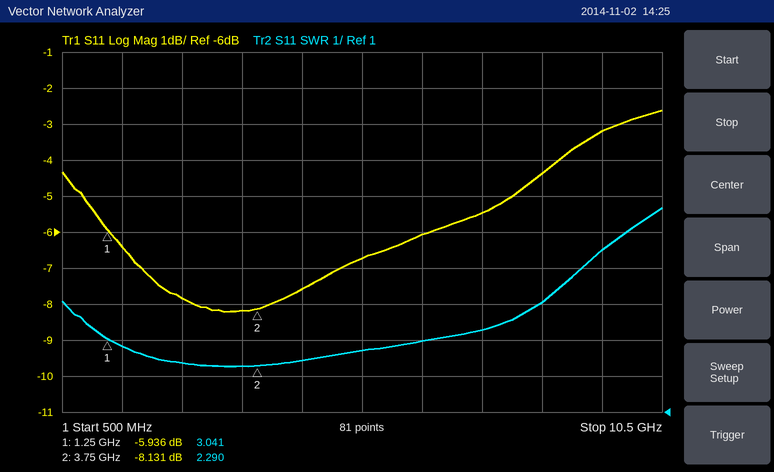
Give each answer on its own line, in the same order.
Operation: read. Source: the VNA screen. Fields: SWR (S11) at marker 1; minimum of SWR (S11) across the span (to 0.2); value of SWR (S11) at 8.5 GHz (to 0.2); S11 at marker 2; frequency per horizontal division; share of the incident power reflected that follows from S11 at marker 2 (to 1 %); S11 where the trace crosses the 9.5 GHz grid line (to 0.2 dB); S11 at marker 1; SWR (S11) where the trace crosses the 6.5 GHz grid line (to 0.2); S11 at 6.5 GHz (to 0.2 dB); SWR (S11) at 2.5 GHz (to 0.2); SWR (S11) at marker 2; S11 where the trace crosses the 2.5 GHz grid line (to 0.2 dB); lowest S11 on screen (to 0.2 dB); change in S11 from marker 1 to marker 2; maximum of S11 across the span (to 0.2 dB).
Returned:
3.041
2.2
4.0
-8.131 dB
1 GHz
15 %
-3.2 dB
-5.936 dB
3.0
-6.0 dB
2.4
2.290
-7.8 dB
-8.2 dB
-2.195 dB
-2.6 dB
